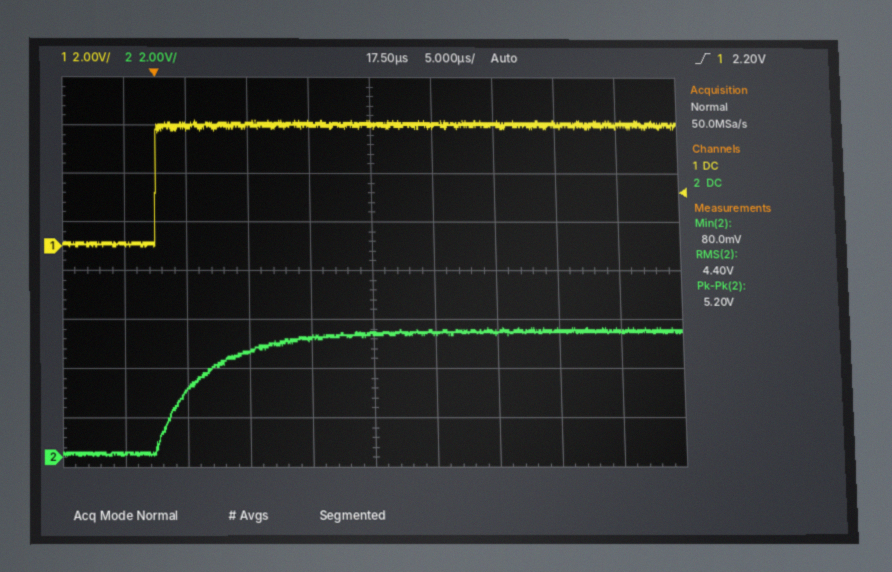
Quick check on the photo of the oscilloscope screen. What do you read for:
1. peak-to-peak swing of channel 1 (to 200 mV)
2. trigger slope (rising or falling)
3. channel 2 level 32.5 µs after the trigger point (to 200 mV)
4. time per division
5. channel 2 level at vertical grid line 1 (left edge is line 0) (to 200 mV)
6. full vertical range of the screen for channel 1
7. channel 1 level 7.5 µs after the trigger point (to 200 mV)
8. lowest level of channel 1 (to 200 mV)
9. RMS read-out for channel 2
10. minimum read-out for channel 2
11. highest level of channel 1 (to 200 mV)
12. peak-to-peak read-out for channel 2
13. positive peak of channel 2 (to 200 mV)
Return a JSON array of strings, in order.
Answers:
["5.2 V", "rising", "5.2 V", "5 µs", "200 mV", "16 V", "5.0 V", "0.0 V", "4.40 V", "80.0 mV", "5.2 V", "5.20 V", "5.2 V"]
